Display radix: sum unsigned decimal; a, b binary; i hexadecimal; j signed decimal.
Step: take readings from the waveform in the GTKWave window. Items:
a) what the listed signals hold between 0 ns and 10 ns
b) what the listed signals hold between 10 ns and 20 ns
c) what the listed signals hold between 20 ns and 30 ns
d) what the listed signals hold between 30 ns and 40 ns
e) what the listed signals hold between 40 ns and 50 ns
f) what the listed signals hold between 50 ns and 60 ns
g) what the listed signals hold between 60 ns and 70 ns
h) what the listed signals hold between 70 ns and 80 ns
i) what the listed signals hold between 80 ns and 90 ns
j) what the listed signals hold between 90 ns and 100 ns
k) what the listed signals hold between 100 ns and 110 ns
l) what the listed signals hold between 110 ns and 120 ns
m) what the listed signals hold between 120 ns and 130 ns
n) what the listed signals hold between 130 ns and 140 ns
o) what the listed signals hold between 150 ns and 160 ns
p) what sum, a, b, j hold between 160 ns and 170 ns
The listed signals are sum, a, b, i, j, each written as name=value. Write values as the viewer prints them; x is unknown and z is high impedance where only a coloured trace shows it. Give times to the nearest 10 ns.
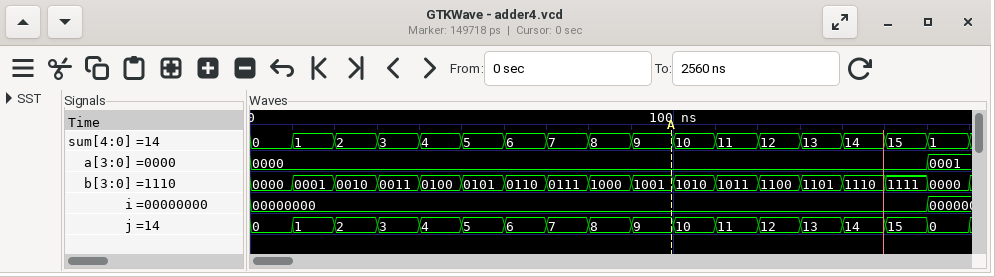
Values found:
sum=0, a=0000, b=0000, i=00000000, j=0
sum=1, a=0000, b=0001, i=00000000, j=1
sum=2, a=0000, b=0010, i=00000000, j=2
sum=3, a=0000, b=0011, i=00000000, j=3
sum=4, a=0000, b=0100, i=00000000, j=4
sum=5, a=0000, b=0101, i=00000000, j=5
sum=6, a=0000, b=0110, i=00000000, j=6
sum=7, a=0000, b=0111, i=00000000, j=7
sum=8, a=0000, b=1000, i=00000000, j=8
sum=9, a=0000, b=1001, i=00000000, j=9
sum=10, a=0000, b=1010, i=00000000, j=10
sum=11, a=0000, b=1011, i=00000000, j=11
sum=12, a=0000, b=1100, i=00000000, j=12
sum=13, a=0000, b=1101, i=00000000, j=13
sum=15, a=0000, b=1111, i=00000000, j=15
sum=1, a=0001, b=0000, j=0
